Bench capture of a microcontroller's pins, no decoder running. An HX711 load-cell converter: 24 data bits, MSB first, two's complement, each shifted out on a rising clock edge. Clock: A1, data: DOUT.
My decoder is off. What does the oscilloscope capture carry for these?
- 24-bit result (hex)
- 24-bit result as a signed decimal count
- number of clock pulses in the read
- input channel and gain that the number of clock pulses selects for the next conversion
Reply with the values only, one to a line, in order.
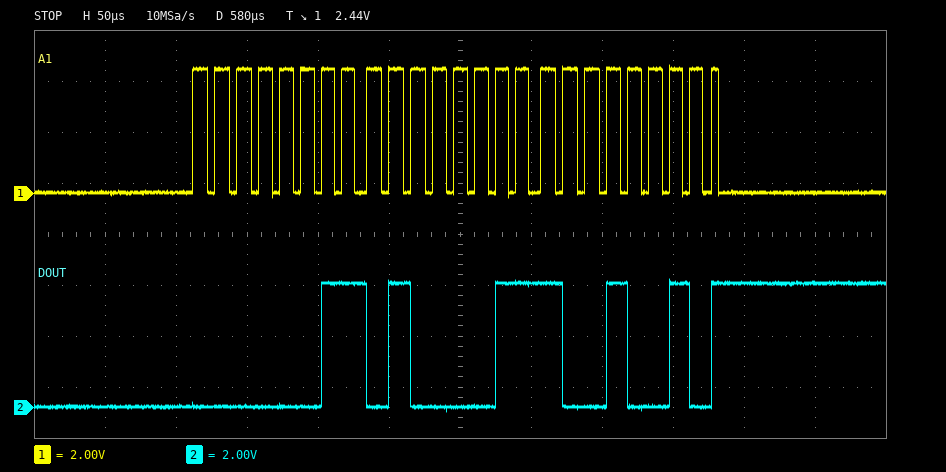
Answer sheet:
0x034392
213906
25
channel A, gain 128
